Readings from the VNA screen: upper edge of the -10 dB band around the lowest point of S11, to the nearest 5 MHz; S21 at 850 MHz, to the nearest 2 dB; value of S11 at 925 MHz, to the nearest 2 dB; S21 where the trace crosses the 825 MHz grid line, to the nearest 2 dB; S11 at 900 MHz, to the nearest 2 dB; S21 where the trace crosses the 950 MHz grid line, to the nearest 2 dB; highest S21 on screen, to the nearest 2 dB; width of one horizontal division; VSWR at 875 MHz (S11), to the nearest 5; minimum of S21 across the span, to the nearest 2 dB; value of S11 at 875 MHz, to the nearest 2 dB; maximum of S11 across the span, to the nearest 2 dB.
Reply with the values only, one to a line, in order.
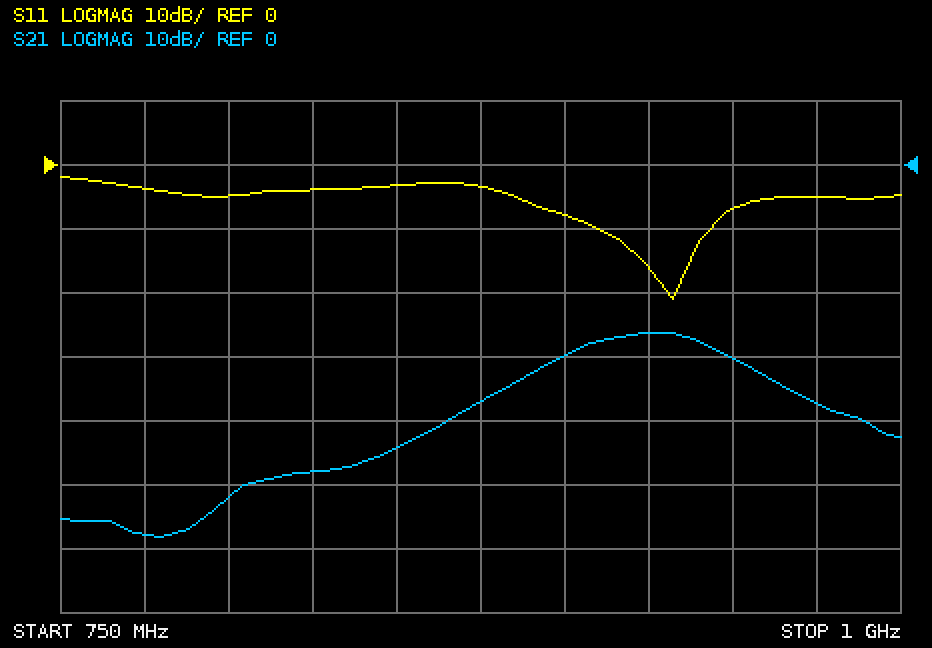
945 MHz
-44 dB
-16 dB
-48 dB
-8 dB
-30 dB
-26 dB
25 MHz
5
-58 dB
-4 dB
-2 dB
